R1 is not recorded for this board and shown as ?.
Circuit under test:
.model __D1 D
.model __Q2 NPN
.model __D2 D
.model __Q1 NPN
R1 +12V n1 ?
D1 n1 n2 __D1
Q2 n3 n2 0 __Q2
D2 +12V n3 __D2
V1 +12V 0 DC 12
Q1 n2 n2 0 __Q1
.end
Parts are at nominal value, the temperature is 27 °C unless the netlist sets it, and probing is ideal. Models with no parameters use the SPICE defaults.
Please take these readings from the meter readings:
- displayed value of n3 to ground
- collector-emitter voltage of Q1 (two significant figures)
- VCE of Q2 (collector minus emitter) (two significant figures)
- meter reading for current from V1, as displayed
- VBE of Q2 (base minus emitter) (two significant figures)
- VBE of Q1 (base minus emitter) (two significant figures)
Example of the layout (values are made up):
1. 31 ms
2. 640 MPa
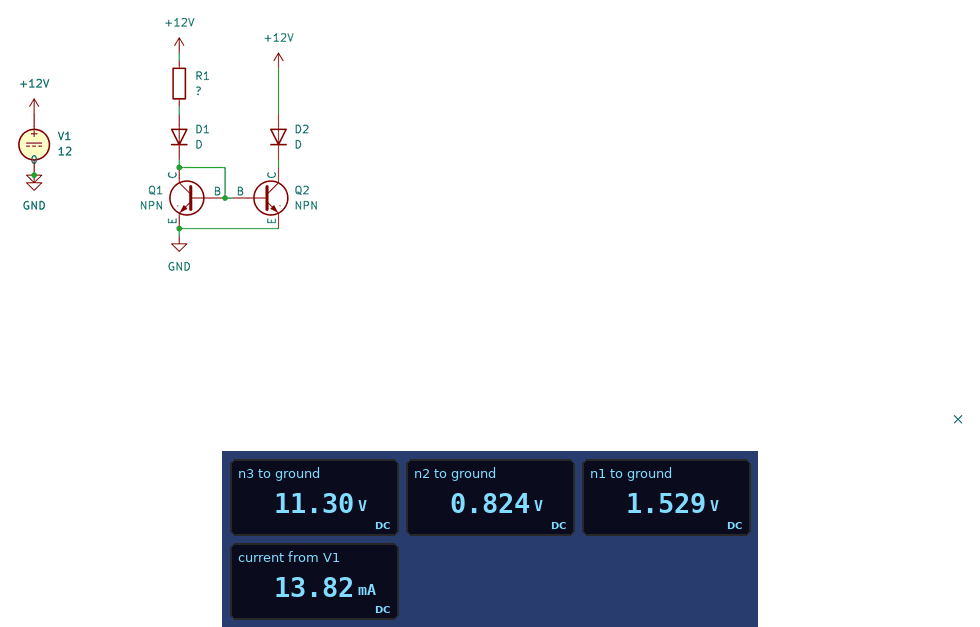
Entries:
1. 11.30 V
2. 820 mV
3. 11 V
4. 13.82 mA
5. 820 mV
6. 820 mV
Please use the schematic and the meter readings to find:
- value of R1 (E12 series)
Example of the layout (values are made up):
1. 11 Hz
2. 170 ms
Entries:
1. 1.5 kΩ
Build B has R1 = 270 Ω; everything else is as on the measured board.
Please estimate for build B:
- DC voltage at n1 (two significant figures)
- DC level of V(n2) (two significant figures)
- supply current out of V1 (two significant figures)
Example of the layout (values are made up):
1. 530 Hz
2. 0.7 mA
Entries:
1. 1.6 V
2. 870 mV
3. 76 mA
